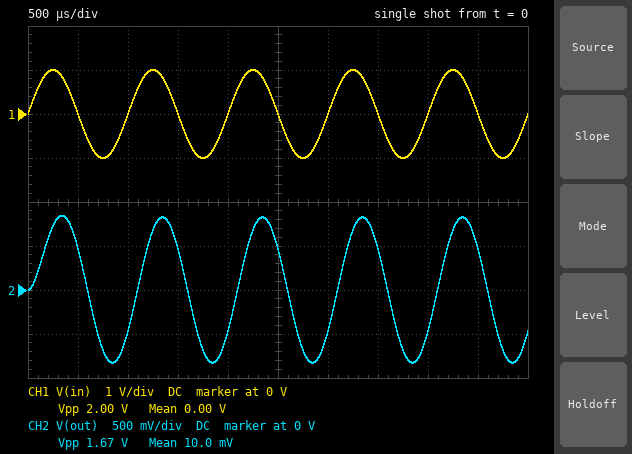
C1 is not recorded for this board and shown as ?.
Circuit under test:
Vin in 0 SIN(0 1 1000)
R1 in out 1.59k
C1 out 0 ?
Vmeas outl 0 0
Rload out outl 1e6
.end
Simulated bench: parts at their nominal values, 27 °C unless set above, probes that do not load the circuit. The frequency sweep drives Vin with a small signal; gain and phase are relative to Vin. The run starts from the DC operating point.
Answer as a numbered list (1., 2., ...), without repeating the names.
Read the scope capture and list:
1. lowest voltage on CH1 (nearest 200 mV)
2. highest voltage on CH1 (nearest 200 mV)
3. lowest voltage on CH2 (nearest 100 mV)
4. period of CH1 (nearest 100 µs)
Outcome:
1. -1.0 V
2. 1.0 V
3. -800 mV
4. 1.0 ms
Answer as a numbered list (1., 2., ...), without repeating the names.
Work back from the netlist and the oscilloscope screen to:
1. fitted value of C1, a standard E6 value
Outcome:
1. 68 nF
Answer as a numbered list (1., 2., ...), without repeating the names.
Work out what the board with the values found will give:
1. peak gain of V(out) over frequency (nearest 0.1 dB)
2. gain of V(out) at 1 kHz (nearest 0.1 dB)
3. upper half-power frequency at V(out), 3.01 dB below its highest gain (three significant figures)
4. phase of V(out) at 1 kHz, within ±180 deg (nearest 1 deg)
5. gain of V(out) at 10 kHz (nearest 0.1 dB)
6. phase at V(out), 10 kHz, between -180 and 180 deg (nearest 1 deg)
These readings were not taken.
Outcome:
1. 0 dB
2. -1.7 dB
3. 1.47 kHz
4. -34 deg
5. -16.7 dB
6. -82 deg
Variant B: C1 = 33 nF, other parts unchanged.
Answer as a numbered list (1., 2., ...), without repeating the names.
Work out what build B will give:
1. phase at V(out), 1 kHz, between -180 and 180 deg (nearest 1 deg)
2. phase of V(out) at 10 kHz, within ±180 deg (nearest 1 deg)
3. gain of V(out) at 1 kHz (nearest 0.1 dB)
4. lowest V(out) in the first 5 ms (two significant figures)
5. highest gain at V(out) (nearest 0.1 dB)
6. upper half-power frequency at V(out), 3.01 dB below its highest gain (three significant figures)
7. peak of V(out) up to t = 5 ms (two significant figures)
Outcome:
1. -18 deg
2. -73 deg
3. -0.5 dB
4. -950 mV
5. 0 dB
6. 3.04 kHz
7. 950 mV
